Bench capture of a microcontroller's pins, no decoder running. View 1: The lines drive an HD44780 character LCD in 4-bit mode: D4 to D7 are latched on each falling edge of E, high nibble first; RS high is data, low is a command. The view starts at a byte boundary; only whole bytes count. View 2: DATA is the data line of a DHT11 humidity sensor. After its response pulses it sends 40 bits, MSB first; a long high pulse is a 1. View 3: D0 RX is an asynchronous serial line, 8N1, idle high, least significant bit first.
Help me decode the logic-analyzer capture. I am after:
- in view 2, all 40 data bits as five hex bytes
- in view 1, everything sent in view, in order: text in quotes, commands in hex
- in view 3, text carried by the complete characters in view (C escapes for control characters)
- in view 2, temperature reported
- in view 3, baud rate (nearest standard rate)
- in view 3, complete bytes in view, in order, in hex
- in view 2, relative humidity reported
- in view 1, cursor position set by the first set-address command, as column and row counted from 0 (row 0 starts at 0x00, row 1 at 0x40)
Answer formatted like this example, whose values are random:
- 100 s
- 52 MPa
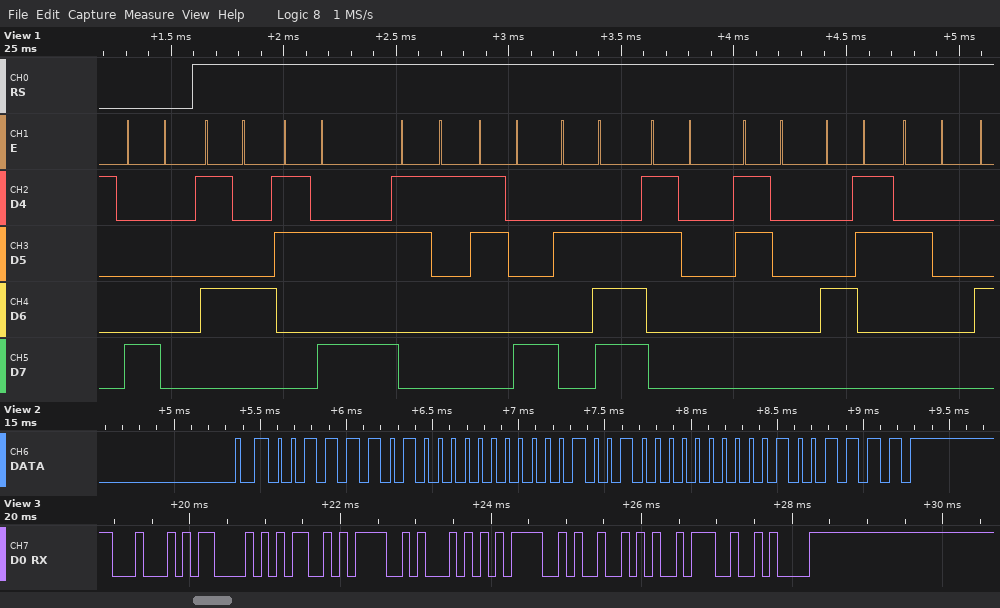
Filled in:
- 3D 00 12 00 4F
- 0x80 "T:18.00C "
- "DCMOTOR:\n"
- 18.0 °C
- 9600 baud
- 44 43 4D 4F 54 4F 52 3A 0A
- 61 %
- column 0, row 0
